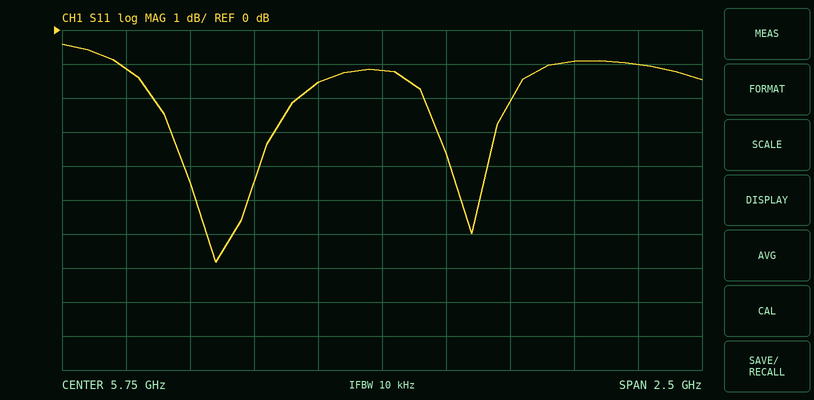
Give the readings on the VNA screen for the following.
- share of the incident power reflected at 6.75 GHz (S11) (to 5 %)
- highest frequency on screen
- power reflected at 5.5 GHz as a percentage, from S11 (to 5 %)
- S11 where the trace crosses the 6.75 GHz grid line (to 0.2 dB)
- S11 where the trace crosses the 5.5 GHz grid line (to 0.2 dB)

80 %
7 GHz
70 %
-1.0 dB
-1.6 dB
